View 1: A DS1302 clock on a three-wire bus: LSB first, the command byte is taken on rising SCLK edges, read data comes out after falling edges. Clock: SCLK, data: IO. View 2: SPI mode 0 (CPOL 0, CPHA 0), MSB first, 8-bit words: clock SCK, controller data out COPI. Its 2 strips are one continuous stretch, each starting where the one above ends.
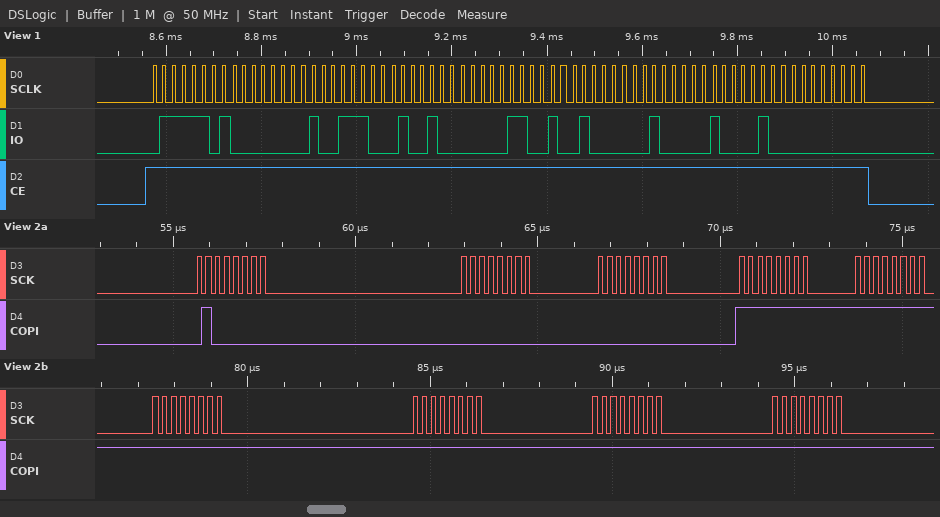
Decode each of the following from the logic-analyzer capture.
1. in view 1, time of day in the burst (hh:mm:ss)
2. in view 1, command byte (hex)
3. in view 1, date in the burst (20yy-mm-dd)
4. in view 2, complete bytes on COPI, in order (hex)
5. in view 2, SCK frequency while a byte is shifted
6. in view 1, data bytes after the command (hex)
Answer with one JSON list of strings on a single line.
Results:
["12:39:00", "0xBE", "2021-09-30", "40 00 00 FF FF FF FF FF FF", "4 MHz", "00 39 12 30 09 04 21 00"]
